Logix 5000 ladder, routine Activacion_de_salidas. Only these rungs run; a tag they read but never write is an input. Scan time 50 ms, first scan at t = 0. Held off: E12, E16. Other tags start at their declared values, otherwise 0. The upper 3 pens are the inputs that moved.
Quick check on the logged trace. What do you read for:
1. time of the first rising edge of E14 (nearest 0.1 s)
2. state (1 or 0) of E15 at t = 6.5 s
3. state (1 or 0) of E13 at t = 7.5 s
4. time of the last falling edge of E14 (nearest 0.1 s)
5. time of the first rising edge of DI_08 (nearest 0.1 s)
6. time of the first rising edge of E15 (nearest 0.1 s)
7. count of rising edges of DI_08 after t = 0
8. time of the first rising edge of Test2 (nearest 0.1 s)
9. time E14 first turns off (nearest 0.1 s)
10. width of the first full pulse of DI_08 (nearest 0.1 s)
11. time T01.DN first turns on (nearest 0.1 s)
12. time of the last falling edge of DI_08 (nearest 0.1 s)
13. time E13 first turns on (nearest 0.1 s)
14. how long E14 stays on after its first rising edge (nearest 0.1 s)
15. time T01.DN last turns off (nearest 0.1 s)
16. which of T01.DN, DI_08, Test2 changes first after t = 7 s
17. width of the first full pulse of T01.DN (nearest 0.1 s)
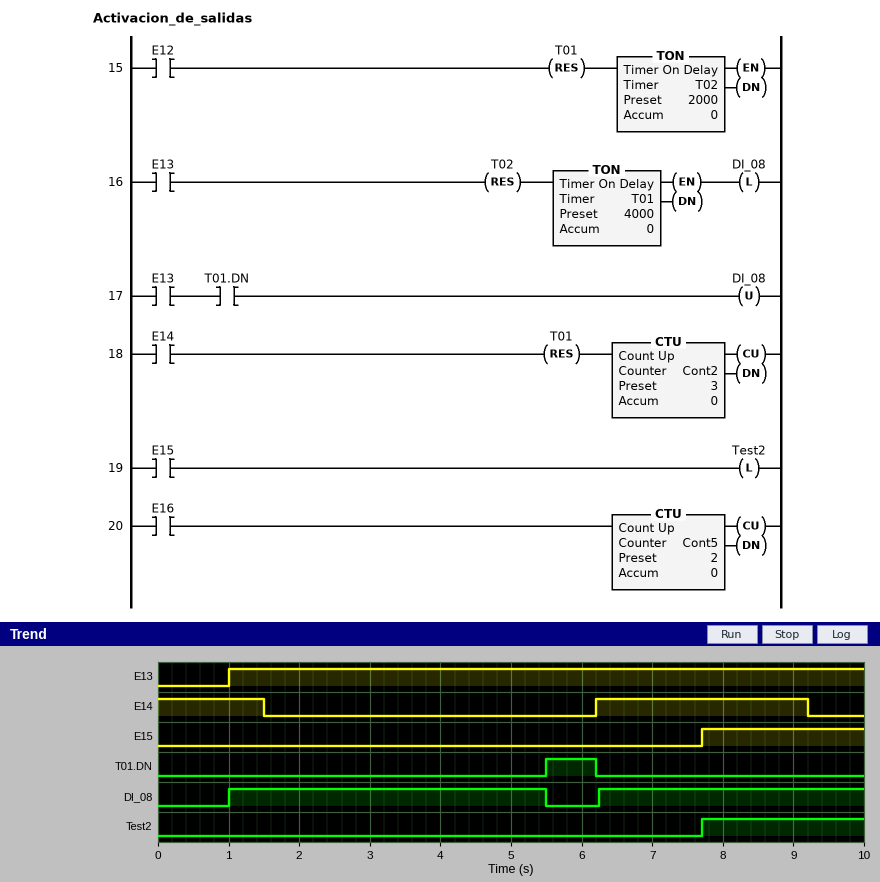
6.2 s
0
1
9.2 s
1.0 s
7.7 s
2
7.7 s
1.5 s
4.5 s
5.5 s
5.5 s
1.0 s
3.0 s
6.2 s
Test2
0.7 s
